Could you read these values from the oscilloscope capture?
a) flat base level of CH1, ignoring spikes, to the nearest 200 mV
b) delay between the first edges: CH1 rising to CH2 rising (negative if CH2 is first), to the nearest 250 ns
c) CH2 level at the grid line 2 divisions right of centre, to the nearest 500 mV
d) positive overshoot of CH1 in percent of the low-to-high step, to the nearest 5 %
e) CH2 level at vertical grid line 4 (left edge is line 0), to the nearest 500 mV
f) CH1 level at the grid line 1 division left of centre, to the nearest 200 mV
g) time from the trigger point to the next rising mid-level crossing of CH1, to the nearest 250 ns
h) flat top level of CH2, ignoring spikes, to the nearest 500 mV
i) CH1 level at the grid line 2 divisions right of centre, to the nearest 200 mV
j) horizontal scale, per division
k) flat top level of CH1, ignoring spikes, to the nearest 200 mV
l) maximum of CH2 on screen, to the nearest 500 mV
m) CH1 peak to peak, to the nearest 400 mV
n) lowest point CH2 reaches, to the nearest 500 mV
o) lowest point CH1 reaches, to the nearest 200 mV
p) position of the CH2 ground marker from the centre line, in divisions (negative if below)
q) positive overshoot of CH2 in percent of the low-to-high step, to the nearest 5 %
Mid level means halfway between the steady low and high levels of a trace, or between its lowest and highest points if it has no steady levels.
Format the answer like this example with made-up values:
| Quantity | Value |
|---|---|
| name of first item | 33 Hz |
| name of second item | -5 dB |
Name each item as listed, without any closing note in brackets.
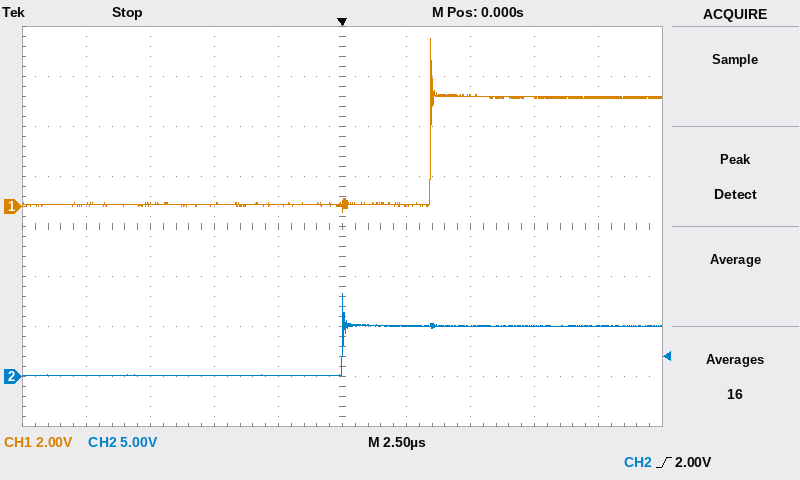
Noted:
| Quantity | Value |
|---|---|
| flat base level of CH1, ignoring spikes, to the nearest 200 mV | 0.0 V |
| delay between the first edges: CH1 rising to CH2 rising (negative if CH2 is first), to the nearest 250 ns | -3.50 µs |
| CH2 level at the grid line 2 divisions right of centre, to the nearest 500 mV | 5.0 V |
| positive overshoot of CH1 in percent of the low-to-high step, to the nearest 5 % | 55 % |
| CH2 level at vertical grid line 4 (left edge is line 0), to the nearest 500 mV | 0.0 V |
| CH1 level at the grid line 1 division left of centre, to the nearest 200 mV | 0.0 V |
| time from the trigger point to the next rising mid-level crossing of CH1, to the nearest 250 ns | 3.50 µs |
| flat top level of CH2, ignoring spikes, to the nearest 500 mV | 5.0 V |
| CH1 level at the grid line 2 divisions right of centre, to the nearest 200 mV | 4.4 V |
| horizontal scale, per division | 2.5 µs |
| flat top level of CH1, ignoring spikes, to the nearest 200 mV | 4.4 V |
| maximum of CH2 on screen, to the nearest 500 mV | 8.5 V |
| CH1 peak to peak, to the nearest 400 mV | 6.8 V |
| lowest point CH2 reaches, to the nearest 500 mV | 0.0 V |
| lowest point CH1 reaches, to the nearest 200 mV | -200 mV |
| position of the CH2 ground marker from the centre line, in divisions | -3.0 div |
| positive overshoot of CH2 in percent of the low-to-high step, to the nearest 5 % | 65 % |
